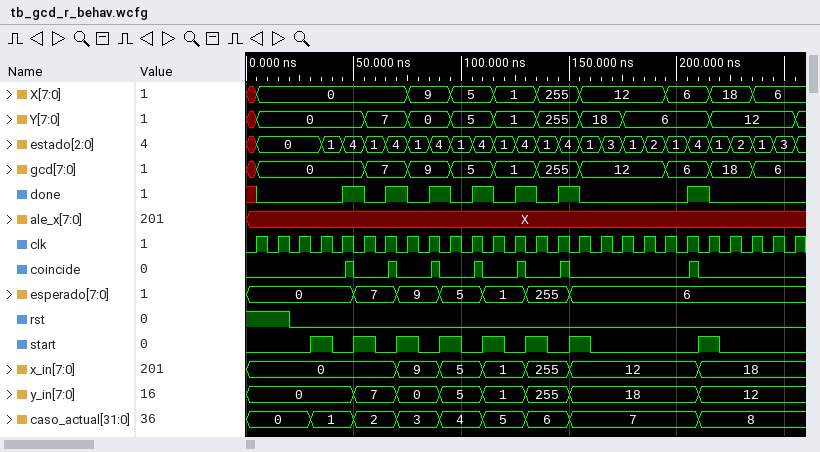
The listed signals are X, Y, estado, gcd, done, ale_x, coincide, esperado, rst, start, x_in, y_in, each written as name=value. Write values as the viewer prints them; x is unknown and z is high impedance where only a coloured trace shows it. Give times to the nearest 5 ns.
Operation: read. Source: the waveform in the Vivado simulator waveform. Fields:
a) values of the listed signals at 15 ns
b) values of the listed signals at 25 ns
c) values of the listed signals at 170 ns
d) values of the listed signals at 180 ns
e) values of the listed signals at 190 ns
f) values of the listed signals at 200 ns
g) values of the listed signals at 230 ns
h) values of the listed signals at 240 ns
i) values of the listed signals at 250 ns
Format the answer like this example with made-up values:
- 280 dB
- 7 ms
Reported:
- X=0, Y=0, estado=0, gcd=0, done=0, ale_x=X, coincide=0, esperado=0, rst=1, start=0, x_in=0, y_in=0
- X=0, Y=0, estado=0, gcd=0, done=0, ale_x=X, coincide=0, esperado=0, rst=0, start=0, x_in=0, y_in=0
- X=12, Y=18, estado=3, gcd=12, done=0, ale_x=X, coincide=0, esperado=6, rst=0, start=0, x_in=12, y_in=18
- X=12, Y=6, estado=1, gcd=12, done=0, ale_x=X, coincide=0, esperado=6, rst=0, start=0, x_in=12, y_in=18
- X=12, Y=6, estado=2, gcd=12, done=0, ale_x=X, coincide=0, esperado=6, rst=0, start=0, x_in=12, y_in=18
- X=6, Y=6, estado=1, gcd=6, done=0, ale_x=X, coincide=0, esperado=6, rst=0, start=0, x_in=12, y_in=18
- X=18, Y=12, estado=2, gcd=18, done=0, ale_x=X, coincide=0, esperado=6, rst=0, start=0, x_in=18, y_in=12
- X=6, Y=12, estado=1, gcd=6, done=0, ale_x=X, coincide=0, esperado=6, rst=0, start=0, x_in=18, y_in=12
- X=6, Y=12, estado=3, gcd=6, done=0, ale_x=X, coincide=0, esperado=6, rst=0, start=0, x_in=18, y_in=12
